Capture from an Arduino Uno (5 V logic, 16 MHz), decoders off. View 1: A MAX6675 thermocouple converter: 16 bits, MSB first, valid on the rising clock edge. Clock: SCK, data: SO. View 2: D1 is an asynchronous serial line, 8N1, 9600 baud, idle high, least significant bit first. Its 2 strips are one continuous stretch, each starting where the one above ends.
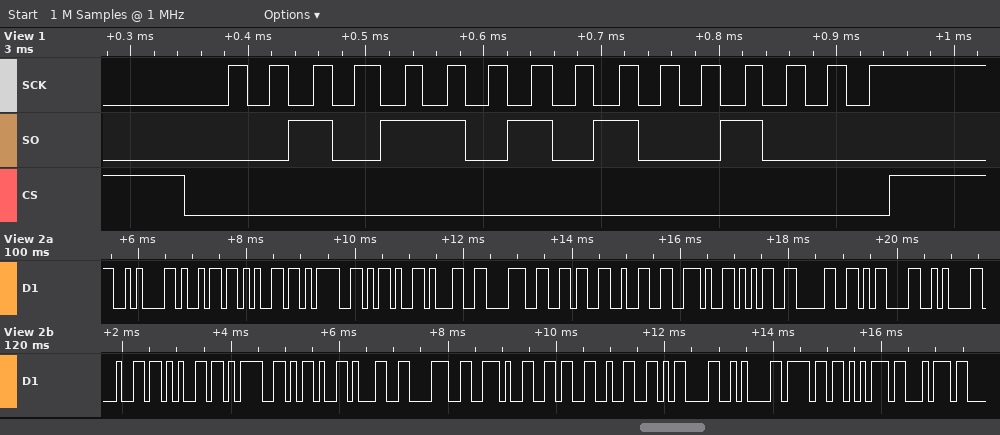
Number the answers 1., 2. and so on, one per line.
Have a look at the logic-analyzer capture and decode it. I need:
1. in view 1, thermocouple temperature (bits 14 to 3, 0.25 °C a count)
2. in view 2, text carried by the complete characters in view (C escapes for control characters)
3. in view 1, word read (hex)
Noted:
1. 362.25 °C
2. "\nie=-1862.50\r\nde=-18.62\r\nout"
3. 0x2D48
